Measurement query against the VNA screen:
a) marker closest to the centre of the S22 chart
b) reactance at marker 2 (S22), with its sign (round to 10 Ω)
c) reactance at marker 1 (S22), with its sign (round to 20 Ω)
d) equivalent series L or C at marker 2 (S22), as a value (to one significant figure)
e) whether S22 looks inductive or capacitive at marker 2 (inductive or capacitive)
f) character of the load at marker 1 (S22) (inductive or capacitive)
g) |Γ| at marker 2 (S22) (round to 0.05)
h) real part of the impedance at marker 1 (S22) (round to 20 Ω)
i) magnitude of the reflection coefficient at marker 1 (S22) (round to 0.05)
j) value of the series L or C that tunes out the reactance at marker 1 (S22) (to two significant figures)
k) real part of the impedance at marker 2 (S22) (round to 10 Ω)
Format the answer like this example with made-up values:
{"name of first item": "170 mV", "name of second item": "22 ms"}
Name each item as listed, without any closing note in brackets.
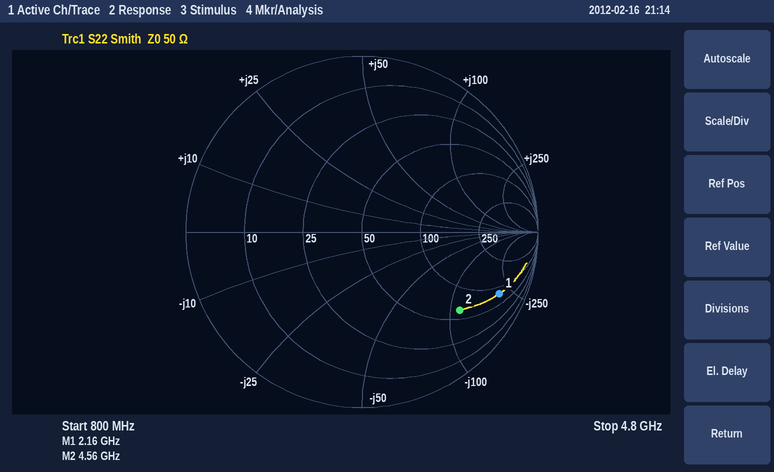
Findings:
{"marker closest to the centre of the S22 chart": "marker 2", "reactance at marker 2 (S22), with its sign": "-110 Ω", "reactance at marker 1 (S22), with its sign": "-200 Ω", "equivalent series L or C at marker 2 (S22), as a value": "300 fF", "whether S22 looks inductive or capacitive at marker 2": "capacitive", "character of the load at marker 1 (S22)": "capacitive", "|Γ| at marker 2 (S22)": "0.70", "real part of the impedance at marker 1 (S22)": "80 Ω", "magnitude of the reflection coefficient at marker 1 (S22)": "0.85", "value of the series L or C that tunes out the reactance at marker 1 (S22)": "15 nH", "real part of the impedance at marker 2 (S22)": "60 Ω"}
